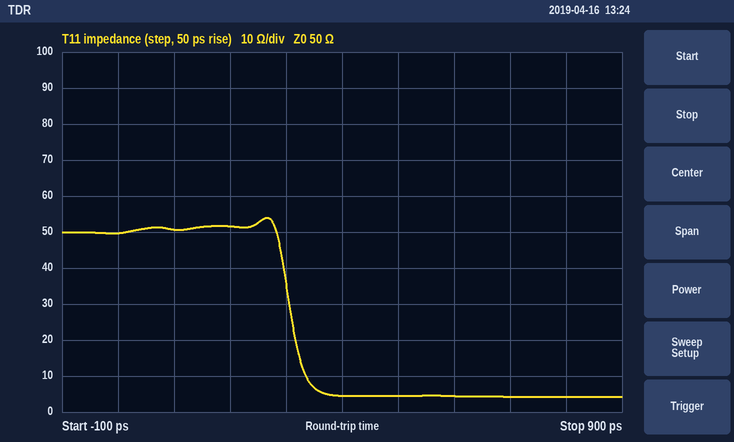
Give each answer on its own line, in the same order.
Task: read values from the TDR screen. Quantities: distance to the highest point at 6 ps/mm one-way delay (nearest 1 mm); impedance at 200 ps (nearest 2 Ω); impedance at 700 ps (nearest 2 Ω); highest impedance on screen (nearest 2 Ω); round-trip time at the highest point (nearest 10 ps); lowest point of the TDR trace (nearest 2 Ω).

22 mm
52 Ω
4 Ω
54 Ω
270 ps
4 Ω
